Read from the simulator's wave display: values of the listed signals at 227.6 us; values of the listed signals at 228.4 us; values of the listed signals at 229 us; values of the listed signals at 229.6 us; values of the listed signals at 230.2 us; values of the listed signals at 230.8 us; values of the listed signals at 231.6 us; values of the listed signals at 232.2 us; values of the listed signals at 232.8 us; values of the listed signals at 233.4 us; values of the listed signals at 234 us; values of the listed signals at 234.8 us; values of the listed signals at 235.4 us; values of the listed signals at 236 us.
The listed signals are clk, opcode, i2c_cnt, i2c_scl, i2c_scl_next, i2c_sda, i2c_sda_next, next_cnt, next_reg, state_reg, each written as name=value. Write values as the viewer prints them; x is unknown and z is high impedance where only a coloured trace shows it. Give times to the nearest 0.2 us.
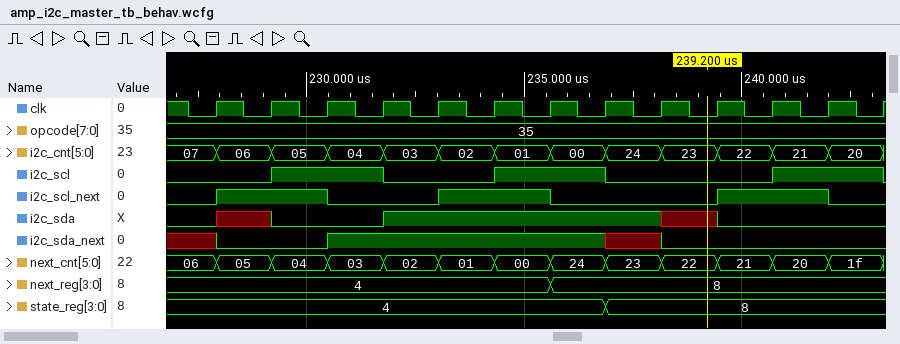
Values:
clk=0, opcode=35, i2c_cnt=07, i2c_scl=0, i2c_scl_next=0, i2c_sda=0, i2c_sda_next=x, next_cnt=06, next_reg=4, state_reg=4
clk=1, opcode=35, i2c_cnt=06, i2c_scl=0, i2c_scl_next=1, i2c_sda=x, i2c_sda_next=0, next_cnt=05, next_reg=4, state_reg=4
clk=0, opcode=35, i2c_cnt=06, i2c_scl=0, i2c_scl_next=1, i2c_sda=x, i2c_sda_next=0, next_cnt=05, next_reg=4, state_reg=4
clk=1, opcode=35, i2c_cnt=05, i2c_scl=1, i2c_scl_next=1, i2c_sda=0, i2c_sda_next=0, next_cnt=04, next_reg=4, state_reg=4
clk=0, opcode=35, i2c_cnt=05, i2c_scl=1, i2c_scl_next=1, i2c_sda=0, i2c_sda_next=0, next_cnt=04, next_reg=4, state_reg=4
clk=1, opcode=35, i2c_cnt=04, i2c_scl=1, i2c_scl_next=0, i2c_sda=0, i2c_sda_next=1, next_cnt=03, next_reg=4, state_reg=4
clk=0, opcode=35, i2c_cnt=04, i2c_scl=1, i2c_scl_next=0, i2c_sda=0, i2c_sda_next=1, next_cnt=03, next_reg=4, state_reg=4
clk=1, opcode=35, i2c_cnt=03, i2c_scl=0, i2c_scl_next=0, i2c_sda=1, i2c_sda_next=1, next_cnt=02, next_reg=4, state_reg=4
clk=0, opcode=35, i2c_cnt=03, i2c_scl=0, i2c_scl_next=0, i2c_sda=1, i2c_sda_next=1, next_cnt=02, next_reg=4, state_reg=4
clk=1, opcode=35, i2c_cnt=02, i2c_scl=0, i2c_scl_next=1, i2c_sda=1, i2c_sda_next=1, next_cnt=01, next_reg=4, state_reg=4
clk=0, opcode=35, i2c_cnt=02, i2c_scl=0, i2c_scl_next=1, i2c_sda=1, i2c_sda_next=1, next_cnt=01, next_reg=4, state_reg=4
clk=1, opcode=35, i2c_cnt=01, i2c_scl=1, i2c_scl_next=1, i2c_sda=1, i2c_sda_next=1, next_cnt=00, next_reg=4, state_reg=4
clk=0, opcode=35, i2c_cnt=01, i2c_scl=1, i2c_scl_next=1, i2c_sda=1, i2c_sda_next=1, next_cnt=00, next_reg=4, state_reg=4
clk=1, opcode=35, i2c_cnt=00, i2c_scl=1, i2c_scl_next=0, i2c_sda=1, i2c_sda_next=1, next_cnt=24, next_reg=8, state_reg=4
